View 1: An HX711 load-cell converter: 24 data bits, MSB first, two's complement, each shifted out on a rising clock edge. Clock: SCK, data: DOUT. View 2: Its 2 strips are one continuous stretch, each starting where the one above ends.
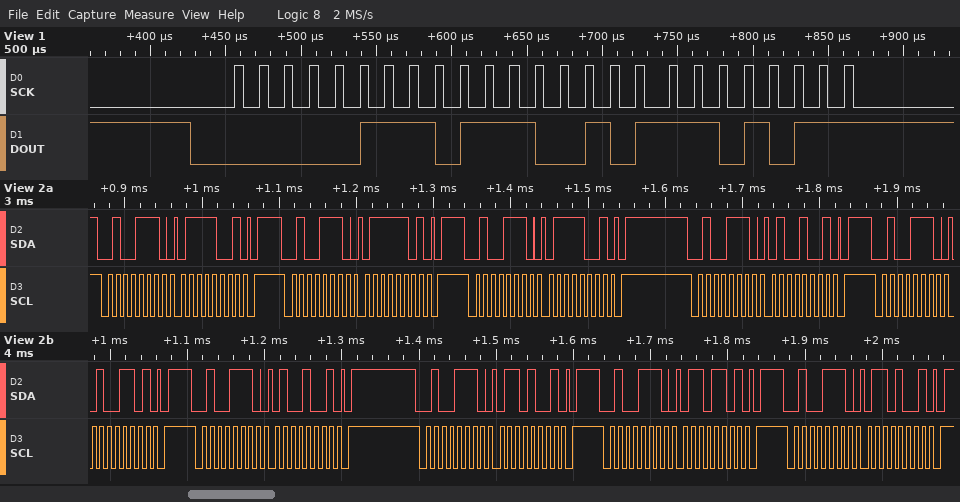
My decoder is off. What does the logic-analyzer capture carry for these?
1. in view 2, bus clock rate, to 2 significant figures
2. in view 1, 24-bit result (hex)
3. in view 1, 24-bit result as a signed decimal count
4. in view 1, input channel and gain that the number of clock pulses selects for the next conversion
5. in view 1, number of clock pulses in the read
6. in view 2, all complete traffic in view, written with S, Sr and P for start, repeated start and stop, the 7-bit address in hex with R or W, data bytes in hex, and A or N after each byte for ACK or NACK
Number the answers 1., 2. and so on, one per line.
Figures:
1. 100 kHz
2. 0x0772EB
3. 488171
4. channel A, gain 128
5. 25
6. S 27W A 79 A P S 27W A 7D A P S 27W A 79 A P S 27W A 49 A P S 27W A 4D A P S 27W A 49 A P S 27W A 69 A P S 27W A 6D A P S 27W A 69 A P
